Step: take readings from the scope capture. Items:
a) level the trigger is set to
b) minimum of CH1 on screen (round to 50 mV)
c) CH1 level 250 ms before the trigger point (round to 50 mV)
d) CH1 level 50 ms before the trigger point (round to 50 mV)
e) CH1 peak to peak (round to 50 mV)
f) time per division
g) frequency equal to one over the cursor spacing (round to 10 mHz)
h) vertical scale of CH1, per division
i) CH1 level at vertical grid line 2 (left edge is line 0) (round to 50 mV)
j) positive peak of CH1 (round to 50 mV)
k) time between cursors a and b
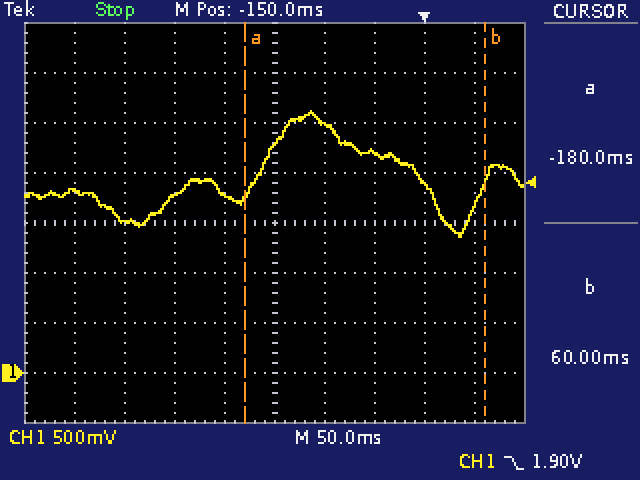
1.90 V
1.35 V
1.80 V
2.20 V
1.25 V
50 ms
4.17 Hz
500 mV
1.50 V
2.60 V
240 ms
